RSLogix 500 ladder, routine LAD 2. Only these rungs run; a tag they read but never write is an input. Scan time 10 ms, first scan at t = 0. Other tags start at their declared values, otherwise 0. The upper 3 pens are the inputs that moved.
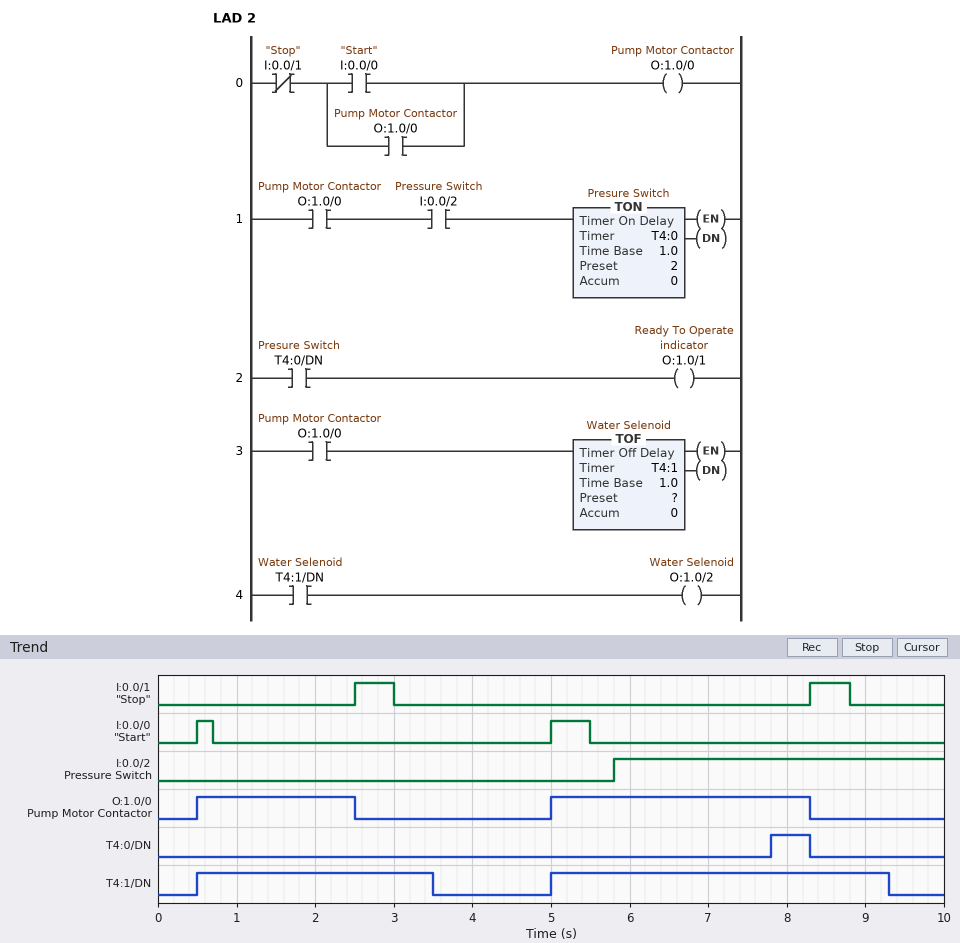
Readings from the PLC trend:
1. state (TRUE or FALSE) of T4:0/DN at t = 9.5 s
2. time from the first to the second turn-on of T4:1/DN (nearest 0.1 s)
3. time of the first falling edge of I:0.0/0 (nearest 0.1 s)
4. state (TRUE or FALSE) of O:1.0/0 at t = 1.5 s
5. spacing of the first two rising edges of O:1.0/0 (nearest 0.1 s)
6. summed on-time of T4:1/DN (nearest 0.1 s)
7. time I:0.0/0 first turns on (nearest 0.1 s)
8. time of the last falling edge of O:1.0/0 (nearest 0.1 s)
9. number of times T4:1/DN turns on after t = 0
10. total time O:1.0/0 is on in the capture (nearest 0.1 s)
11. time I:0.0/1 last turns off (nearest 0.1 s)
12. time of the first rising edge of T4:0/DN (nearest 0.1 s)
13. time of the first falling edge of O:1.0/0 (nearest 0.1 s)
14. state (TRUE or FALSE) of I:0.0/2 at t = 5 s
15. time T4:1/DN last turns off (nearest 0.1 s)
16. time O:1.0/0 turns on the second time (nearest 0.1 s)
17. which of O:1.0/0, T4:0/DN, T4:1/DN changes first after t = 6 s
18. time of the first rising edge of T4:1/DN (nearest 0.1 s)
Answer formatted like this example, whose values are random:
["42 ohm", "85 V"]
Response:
["FALSE", "4.5 s", "0.7 s", "TRUE", "4.5 s", "7.3 s", "0.5 s", "8.3 s", "2", "5.3 s", "8.8 s", "7.8 s", "2.5 s", "FALSE", "9.3 s", "5.0 s", "T4:0/DN", "0.5 s"]
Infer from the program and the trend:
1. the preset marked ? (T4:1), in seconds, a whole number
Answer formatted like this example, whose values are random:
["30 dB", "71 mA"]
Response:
["1 s"]
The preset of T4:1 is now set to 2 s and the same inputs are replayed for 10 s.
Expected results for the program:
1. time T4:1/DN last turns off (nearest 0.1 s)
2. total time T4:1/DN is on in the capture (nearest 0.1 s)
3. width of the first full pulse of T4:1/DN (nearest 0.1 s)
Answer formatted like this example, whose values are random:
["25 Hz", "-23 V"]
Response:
["4.5 s", "9.0 s", "4.0 s"]
